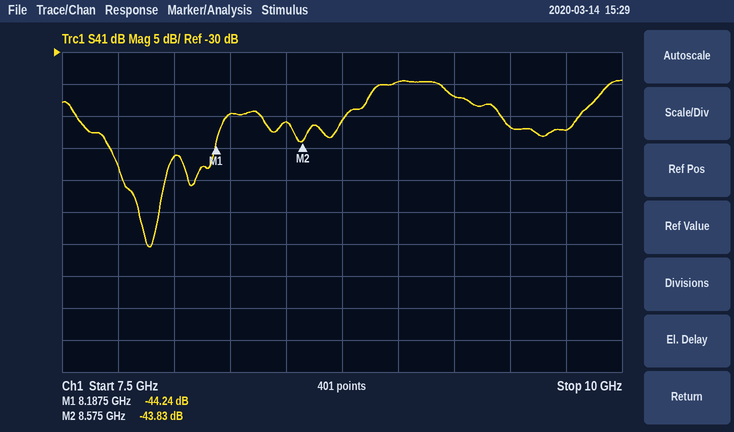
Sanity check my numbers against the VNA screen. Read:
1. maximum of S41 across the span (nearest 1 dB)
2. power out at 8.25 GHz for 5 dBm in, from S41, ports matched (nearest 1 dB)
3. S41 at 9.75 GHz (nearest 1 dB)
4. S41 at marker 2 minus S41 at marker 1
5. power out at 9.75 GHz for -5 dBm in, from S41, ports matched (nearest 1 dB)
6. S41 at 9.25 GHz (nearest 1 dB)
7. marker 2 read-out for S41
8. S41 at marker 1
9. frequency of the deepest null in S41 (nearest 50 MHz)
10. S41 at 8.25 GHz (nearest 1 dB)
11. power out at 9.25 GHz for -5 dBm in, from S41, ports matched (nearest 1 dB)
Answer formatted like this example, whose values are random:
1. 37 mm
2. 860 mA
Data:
1. -34 dB
2. -35 dBm
3. -42 dB
4. 0.41 dB
5. -47 dBm
6. -37 dB
7. -43.83 dB
8. -44.24 dB
9. 7.90 GHz
10. -40 dB
11. -42 dBm
